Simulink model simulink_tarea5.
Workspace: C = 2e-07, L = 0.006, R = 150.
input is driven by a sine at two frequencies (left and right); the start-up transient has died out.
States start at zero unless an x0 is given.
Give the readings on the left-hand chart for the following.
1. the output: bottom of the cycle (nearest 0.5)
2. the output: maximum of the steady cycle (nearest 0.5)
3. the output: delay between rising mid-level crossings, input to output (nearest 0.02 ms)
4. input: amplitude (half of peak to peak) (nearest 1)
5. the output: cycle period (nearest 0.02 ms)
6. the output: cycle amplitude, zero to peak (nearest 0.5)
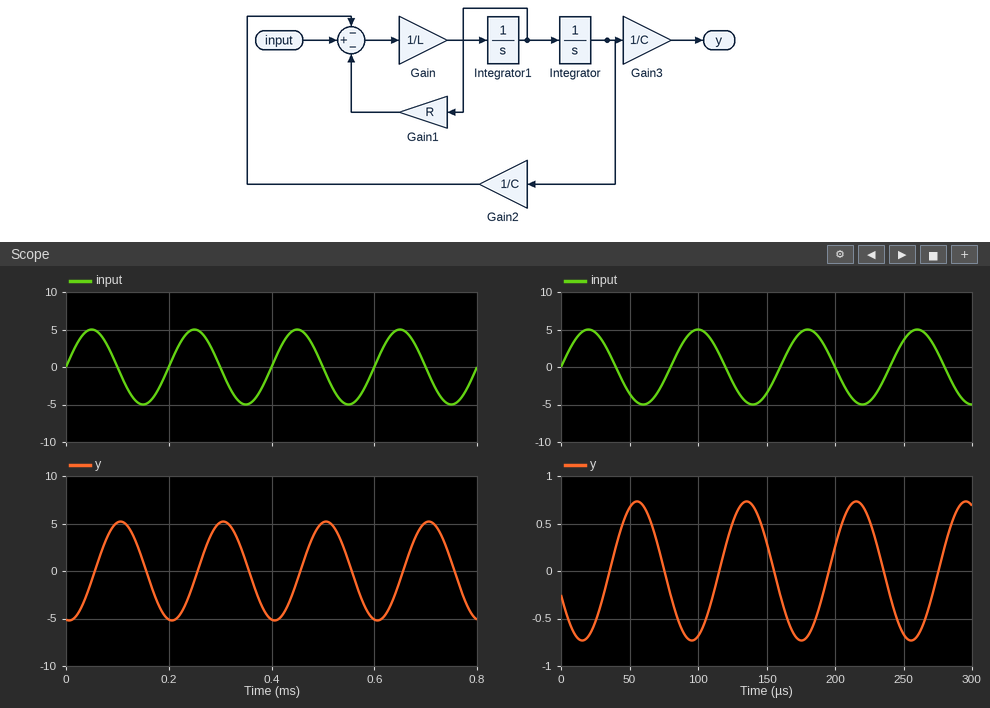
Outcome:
-5.0
5.0
0.06 ms
5
0.20 ms
5.0
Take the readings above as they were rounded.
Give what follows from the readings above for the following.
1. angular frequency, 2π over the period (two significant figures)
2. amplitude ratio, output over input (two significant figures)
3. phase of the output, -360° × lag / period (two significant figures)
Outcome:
31 rad/ms
1.0
-110°
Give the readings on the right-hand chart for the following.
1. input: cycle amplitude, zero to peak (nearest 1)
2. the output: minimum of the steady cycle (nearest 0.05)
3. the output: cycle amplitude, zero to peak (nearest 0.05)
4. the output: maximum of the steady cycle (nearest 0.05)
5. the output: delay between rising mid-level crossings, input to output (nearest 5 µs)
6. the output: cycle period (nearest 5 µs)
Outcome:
5
-0.75
0.75
0.75
35 µs
80 µs
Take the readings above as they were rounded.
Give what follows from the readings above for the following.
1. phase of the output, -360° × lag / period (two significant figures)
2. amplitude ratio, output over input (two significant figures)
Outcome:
-160°
0.15
